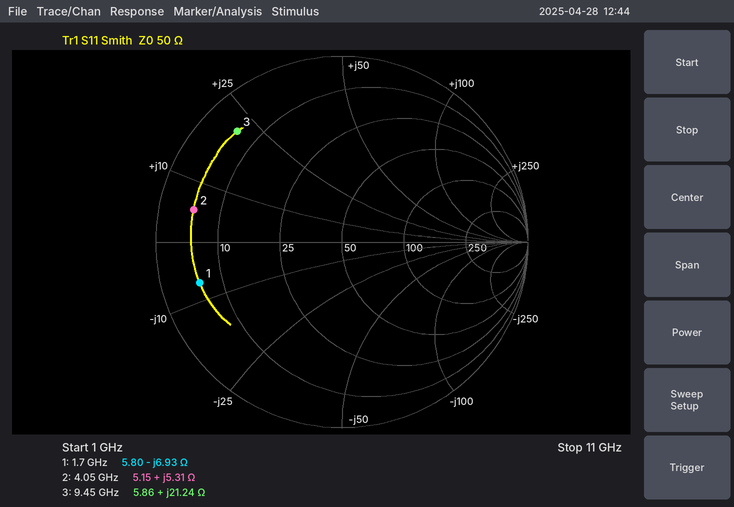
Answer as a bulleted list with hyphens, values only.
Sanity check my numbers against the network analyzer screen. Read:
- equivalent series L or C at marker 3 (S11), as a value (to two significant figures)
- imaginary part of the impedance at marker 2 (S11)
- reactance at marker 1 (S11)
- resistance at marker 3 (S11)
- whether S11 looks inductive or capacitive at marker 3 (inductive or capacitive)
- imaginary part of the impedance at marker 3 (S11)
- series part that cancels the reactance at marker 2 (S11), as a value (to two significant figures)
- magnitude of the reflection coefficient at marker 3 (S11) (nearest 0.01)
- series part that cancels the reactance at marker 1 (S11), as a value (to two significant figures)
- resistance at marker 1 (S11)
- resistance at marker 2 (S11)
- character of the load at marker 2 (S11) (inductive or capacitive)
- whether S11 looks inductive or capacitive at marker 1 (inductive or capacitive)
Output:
- 360 pH
- +5.31 Ω
- -6.93 Ω
- 5.86 Ω
- inductive
- +21.24 Ω
- 7.4 pF
- 0.82
- 650 pH
- 5.80 Ω
- 5.15 Ω
- inductive
- capacitive
